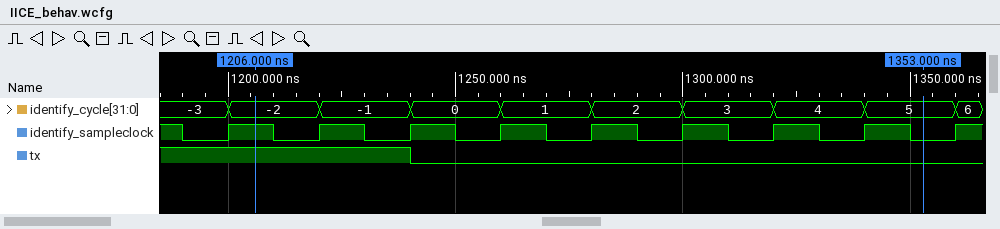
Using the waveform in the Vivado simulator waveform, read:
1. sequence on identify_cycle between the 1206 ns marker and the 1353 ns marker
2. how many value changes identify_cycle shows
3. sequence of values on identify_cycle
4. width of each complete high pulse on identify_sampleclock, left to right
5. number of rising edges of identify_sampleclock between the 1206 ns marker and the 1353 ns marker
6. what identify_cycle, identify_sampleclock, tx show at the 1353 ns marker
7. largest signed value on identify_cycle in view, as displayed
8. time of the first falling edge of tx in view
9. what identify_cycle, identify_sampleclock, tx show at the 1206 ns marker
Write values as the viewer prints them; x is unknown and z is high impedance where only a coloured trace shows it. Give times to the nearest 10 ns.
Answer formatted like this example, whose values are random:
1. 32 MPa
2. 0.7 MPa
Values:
1. -2, -1, 0, 1, 2, 3, 4, 5
2. 9
3. -3, -2, -1, 0, 1, 2, 3, 4, 5, 6
4. 10 ns, 10 ns, 10 ns, 10 ns, 10 ns, 10 ns, 10 ns, 10 ns
5. 7
6. identify_cycle=5, identify_sampleclock=0, tx=0
7. 6
8. 1240 ns
9. identify_cycle=-2, identify_sampleclock=1, tx=1
